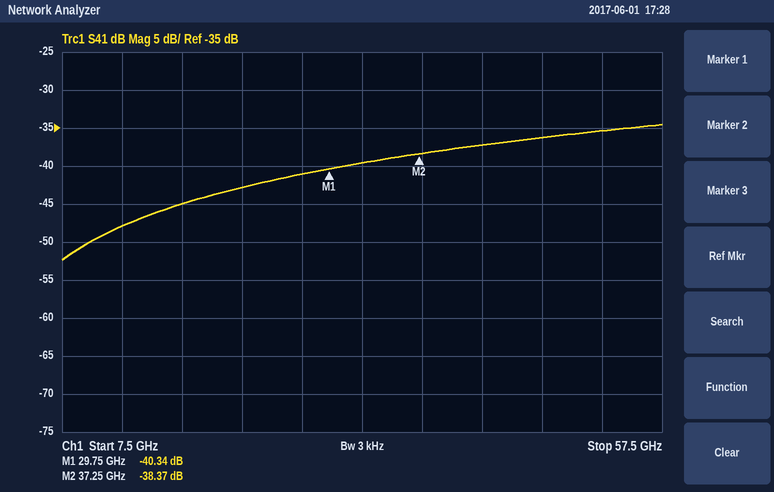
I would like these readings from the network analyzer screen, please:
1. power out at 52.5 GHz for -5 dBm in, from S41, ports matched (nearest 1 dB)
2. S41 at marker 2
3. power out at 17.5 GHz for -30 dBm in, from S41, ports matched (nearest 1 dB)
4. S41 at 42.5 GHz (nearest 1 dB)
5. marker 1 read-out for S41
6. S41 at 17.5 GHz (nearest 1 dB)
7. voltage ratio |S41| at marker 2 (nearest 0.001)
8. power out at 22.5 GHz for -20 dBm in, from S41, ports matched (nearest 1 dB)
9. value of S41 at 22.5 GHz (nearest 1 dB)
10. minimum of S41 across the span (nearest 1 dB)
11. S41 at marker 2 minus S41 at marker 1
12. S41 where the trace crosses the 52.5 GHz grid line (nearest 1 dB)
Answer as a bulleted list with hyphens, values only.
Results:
- -40 dBm
- -38.37 dB
- -75 dBm
- -37 dB
- -40.34 dB
- -45 dB
- 0.012
- -63 dBm
- -43 dB
- -52 dB
- 1.97 dB
- -35 dB
